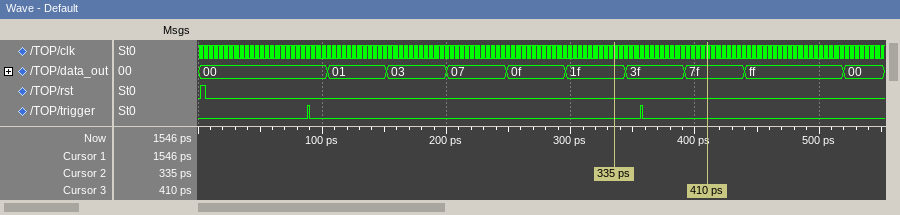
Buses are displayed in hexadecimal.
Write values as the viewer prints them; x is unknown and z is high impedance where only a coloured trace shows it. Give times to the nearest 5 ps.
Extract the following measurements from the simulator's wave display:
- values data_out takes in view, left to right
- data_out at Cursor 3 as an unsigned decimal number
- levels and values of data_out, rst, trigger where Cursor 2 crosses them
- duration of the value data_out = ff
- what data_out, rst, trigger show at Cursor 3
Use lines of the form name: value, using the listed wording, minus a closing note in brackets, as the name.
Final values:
values data_out takes in view, left to right: 00, 01, 03, 07, 0f, 1f, 3f, 7f, ff, 00
data_out at Cursor 3 as an unsigned decimal number: 127
levels and values of data_out, rst, trigger where Cursor 2 crosses them: data_out=1f, rst=0, trigger=0
duration of the value data_out = ff: 80 ps
what data_out, rst, trigger show at Cursor 3: data_out=7f, rst=0, trigger=0
